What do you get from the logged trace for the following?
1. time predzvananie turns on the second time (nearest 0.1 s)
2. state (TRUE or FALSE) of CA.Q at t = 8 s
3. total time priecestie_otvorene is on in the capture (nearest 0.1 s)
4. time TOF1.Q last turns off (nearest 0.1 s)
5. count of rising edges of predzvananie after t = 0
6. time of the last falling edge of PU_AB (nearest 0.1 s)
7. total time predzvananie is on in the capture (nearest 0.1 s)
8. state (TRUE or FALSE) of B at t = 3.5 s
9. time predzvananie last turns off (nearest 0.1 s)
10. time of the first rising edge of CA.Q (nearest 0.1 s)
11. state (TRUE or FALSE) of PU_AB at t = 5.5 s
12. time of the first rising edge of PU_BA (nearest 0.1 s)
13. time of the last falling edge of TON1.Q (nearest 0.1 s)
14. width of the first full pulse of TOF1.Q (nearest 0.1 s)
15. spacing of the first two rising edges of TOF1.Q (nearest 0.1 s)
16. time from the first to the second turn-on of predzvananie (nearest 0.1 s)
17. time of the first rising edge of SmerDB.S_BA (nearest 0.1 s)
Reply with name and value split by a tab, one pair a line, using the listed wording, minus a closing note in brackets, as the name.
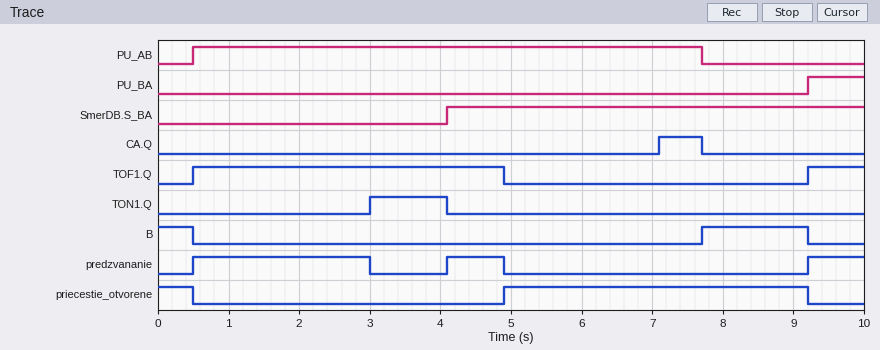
time predzvananie turns on the second time	4.1 s
state (TRUE or FALSE) of CA.Q at t = 8 s	FALSE
total time priecestie_otvorene is on in the capture	4.8 s
time TOF1.Q last turns off	4.9 s
count of rising edges of predzvananie after t = 0	3
time of the last falling edge of PU_AB	7.7 s
total time predzvananie is on in the capture	4.1 s
state (TRUE or FALSE) of B at t = 3.5 s	FALSE
time predzvananie last turns off	4.9 s
time of the first rising edge of CA.Q	7.1 s
state (TRUE or FALSE) of PU_AB at t = 5.5 s	TRUE
time of the first rising edge of PU_BA	9.2 s
time of the last falling edge of TON1.Q	4.1 s
width of the first full pulse of TOF1.Q	4.4 s
spacing of the first two rising edges of TOF1.Q	8.7 s
time from the first to the second turn-on of predzvananie	3.6 s
time of the first rising edge of SmerDB.S_BA	4.1 s
